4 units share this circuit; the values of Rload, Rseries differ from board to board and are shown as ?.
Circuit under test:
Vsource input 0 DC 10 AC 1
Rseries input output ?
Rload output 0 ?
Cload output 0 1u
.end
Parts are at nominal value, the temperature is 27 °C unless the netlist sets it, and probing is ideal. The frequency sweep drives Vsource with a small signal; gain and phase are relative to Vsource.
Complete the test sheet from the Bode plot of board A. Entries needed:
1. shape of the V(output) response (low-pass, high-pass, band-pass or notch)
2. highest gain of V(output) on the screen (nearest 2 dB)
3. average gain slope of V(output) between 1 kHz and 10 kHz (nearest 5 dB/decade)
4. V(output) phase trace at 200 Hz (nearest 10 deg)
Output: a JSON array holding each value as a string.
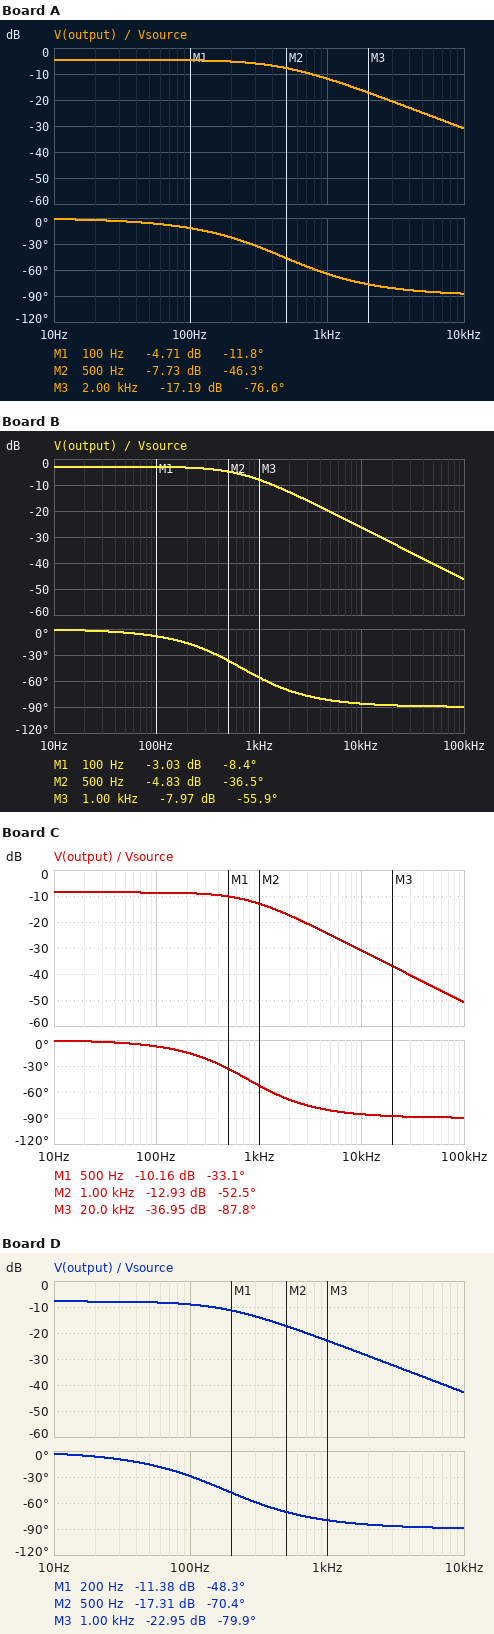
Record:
["low-pass", "-4 dB", "-20 dB/decade", "-20 deg"]
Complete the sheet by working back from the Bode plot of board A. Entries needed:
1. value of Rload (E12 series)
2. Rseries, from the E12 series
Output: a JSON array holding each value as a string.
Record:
["820 Ω", "560 Ω"]
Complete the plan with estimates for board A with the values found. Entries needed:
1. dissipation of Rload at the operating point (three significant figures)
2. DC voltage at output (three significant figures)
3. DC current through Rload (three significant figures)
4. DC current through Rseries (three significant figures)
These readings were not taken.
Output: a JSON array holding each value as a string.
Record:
["43.1 mW", "5.94 V", "7.25 mA", "7.25 mA"]
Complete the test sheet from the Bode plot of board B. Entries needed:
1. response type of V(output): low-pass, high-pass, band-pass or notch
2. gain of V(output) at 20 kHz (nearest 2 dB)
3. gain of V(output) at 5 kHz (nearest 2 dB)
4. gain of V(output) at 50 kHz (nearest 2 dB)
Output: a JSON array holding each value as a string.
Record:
["low-pass", "-32 dB", "-20 dB", "-40 dB"]
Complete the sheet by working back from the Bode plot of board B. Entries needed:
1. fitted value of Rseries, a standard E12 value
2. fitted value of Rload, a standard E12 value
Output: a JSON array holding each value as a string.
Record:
["330 Ω", "820 Ω"]
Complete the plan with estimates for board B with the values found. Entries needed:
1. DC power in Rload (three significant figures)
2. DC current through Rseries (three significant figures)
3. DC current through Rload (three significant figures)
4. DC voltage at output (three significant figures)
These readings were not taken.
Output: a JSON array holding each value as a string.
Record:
["62.0 mW", "8.70 mA", "8.70 mA", "7.13 V"]
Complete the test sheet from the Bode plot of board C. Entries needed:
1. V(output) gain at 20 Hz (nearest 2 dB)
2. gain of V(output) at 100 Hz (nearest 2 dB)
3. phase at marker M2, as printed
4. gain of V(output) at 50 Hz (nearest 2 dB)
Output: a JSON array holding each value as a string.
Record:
["-8 dB", "-8 dB", "-52.5 deg", "-8 dB"]
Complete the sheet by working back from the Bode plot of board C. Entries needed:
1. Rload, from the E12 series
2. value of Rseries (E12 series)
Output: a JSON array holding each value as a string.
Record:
["330 Ω", "560 Ω"]
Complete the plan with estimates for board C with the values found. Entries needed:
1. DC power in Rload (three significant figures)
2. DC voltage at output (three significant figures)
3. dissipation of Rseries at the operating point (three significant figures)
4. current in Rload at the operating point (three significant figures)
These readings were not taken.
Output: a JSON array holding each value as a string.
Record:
["41.7 mW", "3.71 V", "70.7 mW", "11.2 mA"]
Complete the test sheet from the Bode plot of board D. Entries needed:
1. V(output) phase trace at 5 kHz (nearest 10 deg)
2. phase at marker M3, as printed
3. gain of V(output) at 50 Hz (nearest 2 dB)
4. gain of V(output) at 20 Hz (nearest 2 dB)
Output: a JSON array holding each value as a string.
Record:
["-90 deg", "-79.9 deg", "-8 dB", "-8 dB"]
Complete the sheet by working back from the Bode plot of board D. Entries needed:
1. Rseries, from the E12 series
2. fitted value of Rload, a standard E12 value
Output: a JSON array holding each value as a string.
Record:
["2.2 kΩ", "1.5 kΩ"]
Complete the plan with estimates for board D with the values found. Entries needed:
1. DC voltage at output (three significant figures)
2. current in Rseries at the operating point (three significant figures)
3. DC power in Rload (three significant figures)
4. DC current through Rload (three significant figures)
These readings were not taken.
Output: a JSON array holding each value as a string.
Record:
["4.05 V", "2.70 mA", "11.0 mW", "2.70 mA"]
